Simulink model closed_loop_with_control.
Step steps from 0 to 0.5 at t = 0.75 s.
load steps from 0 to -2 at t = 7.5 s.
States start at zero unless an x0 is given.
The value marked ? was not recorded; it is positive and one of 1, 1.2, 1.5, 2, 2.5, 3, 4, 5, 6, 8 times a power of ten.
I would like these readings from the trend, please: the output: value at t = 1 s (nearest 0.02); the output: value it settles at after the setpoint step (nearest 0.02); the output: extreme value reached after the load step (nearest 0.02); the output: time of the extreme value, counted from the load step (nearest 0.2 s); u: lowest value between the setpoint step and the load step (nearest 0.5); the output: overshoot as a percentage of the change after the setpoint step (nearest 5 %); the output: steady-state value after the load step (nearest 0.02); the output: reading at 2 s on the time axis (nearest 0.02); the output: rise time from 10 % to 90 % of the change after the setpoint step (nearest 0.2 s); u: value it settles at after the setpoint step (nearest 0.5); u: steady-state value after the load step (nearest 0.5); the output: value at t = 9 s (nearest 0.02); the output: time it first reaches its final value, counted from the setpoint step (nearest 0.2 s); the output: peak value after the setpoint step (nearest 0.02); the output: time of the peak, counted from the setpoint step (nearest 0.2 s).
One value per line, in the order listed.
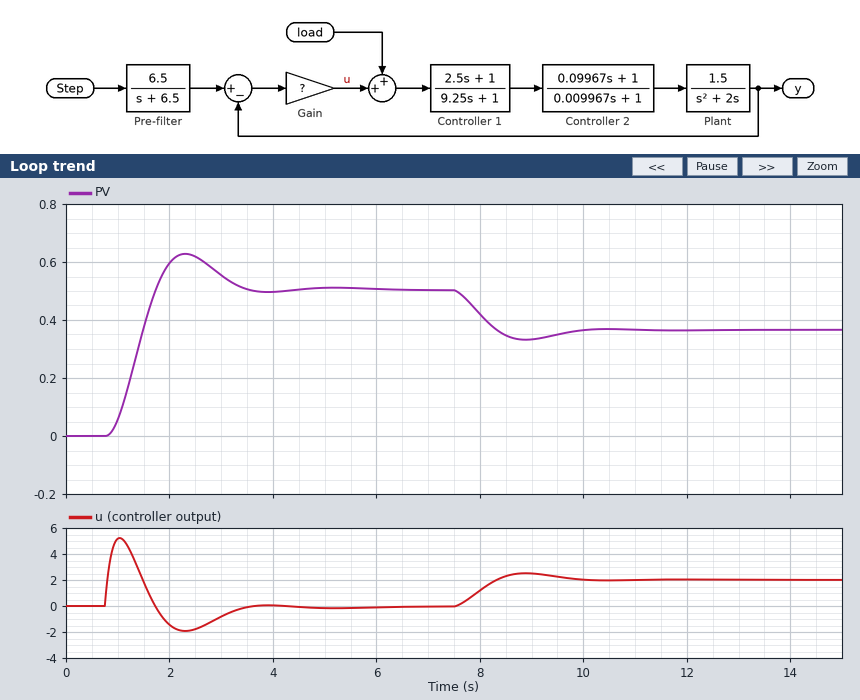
0.06
0.50
0.34
1.4 s
-2.0
25 %
0.36
0.60
0.6 s
0.0
2.0
0.34
1.0 s
0.62
1.6 s
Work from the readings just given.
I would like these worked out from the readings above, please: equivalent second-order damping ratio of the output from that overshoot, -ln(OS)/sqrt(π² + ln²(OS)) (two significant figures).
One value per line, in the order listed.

0.40
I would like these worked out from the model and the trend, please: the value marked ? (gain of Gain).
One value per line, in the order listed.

15
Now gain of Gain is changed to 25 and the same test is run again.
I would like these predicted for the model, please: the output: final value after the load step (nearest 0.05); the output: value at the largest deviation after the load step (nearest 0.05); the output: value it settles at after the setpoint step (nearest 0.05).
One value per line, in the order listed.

0.40
0.40
0.50
